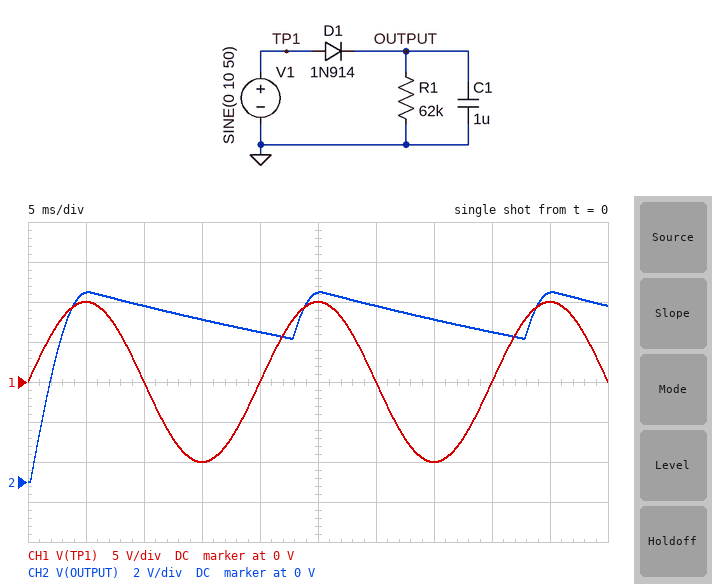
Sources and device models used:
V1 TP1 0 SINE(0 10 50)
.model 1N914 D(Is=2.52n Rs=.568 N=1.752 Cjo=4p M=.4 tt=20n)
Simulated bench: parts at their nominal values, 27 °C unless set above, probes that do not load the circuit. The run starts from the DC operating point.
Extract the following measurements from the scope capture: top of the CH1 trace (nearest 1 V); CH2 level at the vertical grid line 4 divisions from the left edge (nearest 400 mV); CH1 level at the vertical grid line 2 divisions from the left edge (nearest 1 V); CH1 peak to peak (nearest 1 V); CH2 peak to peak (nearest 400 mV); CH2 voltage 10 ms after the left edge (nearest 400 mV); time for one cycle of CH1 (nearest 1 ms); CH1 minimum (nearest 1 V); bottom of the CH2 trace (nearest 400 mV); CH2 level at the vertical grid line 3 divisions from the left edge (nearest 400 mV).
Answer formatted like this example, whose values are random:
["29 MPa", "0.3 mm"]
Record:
["10 V", "7.6 V", "0 V", "20 V", "9.6 V", "8.8 V", "20 ms", "-10 V", "0 V", "8.0 V"]
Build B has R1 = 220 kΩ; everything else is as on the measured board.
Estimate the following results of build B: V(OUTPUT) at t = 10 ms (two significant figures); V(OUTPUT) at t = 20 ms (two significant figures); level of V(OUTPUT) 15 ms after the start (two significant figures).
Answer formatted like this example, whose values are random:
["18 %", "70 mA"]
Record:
["9.3 V", "8.9 V", "9.1 V"]
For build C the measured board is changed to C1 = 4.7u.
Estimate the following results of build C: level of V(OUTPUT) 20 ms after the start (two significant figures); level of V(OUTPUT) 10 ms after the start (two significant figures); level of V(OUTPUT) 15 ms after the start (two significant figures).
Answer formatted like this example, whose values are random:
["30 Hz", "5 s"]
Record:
["9.0 V", "9.3 V", "9.1 V"]
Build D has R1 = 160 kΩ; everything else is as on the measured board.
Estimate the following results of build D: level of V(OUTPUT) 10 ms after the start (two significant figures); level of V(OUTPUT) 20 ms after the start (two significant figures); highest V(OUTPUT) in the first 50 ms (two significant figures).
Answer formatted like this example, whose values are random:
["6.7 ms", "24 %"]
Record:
["9.2 V", "8.7 V", "9.5 V"]
